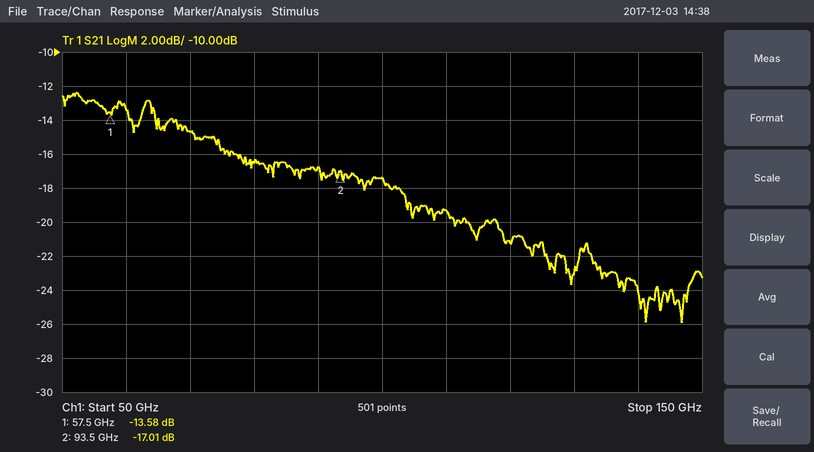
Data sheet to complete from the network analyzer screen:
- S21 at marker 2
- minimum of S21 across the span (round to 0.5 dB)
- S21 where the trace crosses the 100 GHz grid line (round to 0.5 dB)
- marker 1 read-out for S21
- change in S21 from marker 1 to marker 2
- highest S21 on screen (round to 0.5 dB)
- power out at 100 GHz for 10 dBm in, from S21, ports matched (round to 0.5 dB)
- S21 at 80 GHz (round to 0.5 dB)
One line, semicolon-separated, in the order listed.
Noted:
-17.01 dB; -26.0 dB; -17.5 dB; -13.58 dB; -3.43 dB; -12.5 dB; -7.5 dBm; -16.5 dB
